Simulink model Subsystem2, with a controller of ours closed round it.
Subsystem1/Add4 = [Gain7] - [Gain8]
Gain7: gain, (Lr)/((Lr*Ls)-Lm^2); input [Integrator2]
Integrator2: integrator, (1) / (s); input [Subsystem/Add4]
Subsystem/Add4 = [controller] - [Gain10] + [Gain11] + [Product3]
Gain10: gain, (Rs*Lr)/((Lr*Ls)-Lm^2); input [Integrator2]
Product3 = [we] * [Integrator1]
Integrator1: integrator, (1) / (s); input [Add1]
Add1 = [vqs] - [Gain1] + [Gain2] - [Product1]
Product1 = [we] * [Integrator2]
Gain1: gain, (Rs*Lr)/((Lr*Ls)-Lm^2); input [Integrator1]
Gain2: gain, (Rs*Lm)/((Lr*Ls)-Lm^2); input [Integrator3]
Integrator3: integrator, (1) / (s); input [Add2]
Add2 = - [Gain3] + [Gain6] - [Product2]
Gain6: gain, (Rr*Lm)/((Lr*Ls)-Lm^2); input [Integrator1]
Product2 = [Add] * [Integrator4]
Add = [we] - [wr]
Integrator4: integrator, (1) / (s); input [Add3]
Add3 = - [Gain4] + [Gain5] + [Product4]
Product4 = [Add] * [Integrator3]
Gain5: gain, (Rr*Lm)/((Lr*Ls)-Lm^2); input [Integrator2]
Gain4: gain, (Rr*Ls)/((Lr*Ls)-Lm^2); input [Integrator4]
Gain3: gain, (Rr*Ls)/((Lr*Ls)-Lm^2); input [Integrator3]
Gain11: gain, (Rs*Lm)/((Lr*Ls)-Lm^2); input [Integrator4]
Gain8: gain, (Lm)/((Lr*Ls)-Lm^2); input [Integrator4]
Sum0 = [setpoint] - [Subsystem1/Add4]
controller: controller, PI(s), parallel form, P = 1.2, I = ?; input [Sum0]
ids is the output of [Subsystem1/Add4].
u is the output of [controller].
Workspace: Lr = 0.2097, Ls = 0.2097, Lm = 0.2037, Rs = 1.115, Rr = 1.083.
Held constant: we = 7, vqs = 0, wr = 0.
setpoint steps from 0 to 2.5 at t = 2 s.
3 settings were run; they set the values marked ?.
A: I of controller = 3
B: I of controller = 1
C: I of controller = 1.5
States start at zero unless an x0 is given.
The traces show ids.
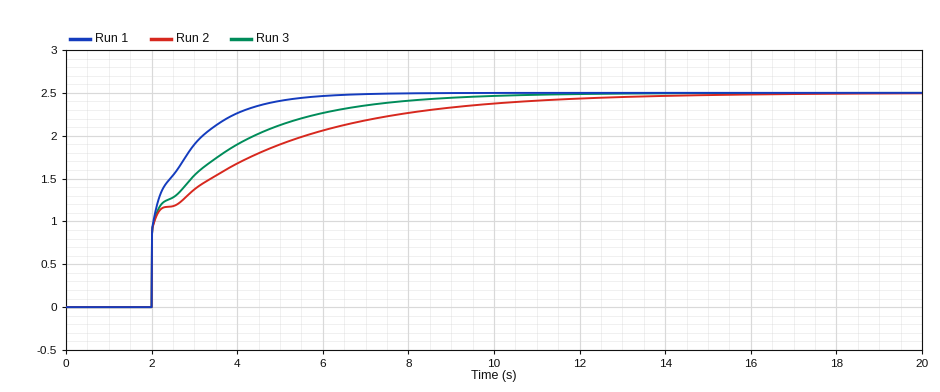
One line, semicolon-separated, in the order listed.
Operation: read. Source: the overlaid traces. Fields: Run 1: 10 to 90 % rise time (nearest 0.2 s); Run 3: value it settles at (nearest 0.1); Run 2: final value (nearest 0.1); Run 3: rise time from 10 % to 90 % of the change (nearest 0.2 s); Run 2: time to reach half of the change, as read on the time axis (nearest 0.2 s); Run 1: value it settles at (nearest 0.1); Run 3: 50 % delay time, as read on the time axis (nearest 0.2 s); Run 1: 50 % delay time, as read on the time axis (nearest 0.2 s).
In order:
2.0 s; 2.5; 2.5; 3.8 s; 2.8 s; 2.5; 2.4 s; 2.2 s
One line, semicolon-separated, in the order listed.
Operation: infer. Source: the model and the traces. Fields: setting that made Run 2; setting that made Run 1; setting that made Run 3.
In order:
B; A; C
